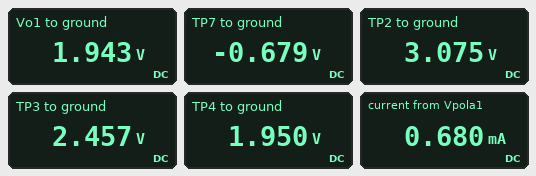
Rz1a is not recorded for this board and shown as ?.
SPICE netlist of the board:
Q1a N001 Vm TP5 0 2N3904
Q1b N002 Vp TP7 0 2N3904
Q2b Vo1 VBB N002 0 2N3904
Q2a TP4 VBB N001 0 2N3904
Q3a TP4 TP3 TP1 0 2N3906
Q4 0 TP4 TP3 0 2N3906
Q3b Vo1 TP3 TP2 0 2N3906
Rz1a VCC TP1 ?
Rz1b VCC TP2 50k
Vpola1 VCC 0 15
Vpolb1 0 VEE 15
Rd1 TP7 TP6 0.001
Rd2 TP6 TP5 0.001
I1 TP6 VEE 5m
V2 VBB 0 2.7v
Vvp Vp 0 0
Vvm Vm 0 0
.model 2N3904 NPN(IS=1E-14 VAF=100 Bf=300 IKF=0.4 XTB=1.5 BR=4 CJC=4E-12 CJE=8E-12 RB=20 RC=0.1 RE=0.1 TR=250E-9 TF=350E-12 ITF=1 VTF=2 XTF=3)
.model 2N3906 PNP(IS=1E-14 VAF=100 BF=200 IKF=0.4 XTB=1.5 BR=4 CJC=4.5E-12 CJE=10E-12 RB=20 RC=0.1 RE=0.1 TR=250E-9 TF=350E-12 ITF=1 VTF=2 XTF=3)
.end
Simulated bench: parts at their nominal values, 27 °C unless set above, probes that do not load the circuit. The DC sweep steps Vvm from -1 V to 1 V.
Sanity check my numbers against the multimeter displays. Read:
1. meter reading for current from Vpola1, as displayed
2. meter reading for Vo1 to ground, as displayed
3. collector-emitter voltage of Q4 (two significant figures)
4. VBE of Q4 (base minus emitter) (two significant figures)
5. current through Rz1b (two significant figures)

0.680 mA
1.943 V
-2.5 V
-510 mV
240 µA
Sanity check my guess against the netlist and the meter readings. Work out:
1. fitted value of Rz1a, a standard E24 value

27 kΩ
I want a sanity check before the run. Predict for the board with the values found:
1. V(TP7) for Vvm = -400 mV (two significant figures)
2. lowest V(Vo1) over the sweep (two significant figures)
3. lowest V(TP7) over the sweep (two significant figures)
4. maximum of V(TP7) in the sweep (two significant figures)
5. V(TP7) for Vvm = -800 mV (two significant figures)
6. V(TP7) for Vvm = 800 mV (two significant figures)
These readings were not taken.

-700 mV
1.9 V
-700 mV
300 mV
-700 mV
100 mV
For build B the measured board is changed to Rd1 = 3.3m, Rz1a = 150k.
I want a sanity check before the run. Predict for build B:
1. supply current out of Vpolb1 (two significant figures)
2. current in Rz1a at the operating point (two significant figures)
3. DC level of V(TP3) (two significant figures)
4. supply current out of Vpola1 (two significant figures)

5.0 mA
80 µA
2.4 V
320 µA
